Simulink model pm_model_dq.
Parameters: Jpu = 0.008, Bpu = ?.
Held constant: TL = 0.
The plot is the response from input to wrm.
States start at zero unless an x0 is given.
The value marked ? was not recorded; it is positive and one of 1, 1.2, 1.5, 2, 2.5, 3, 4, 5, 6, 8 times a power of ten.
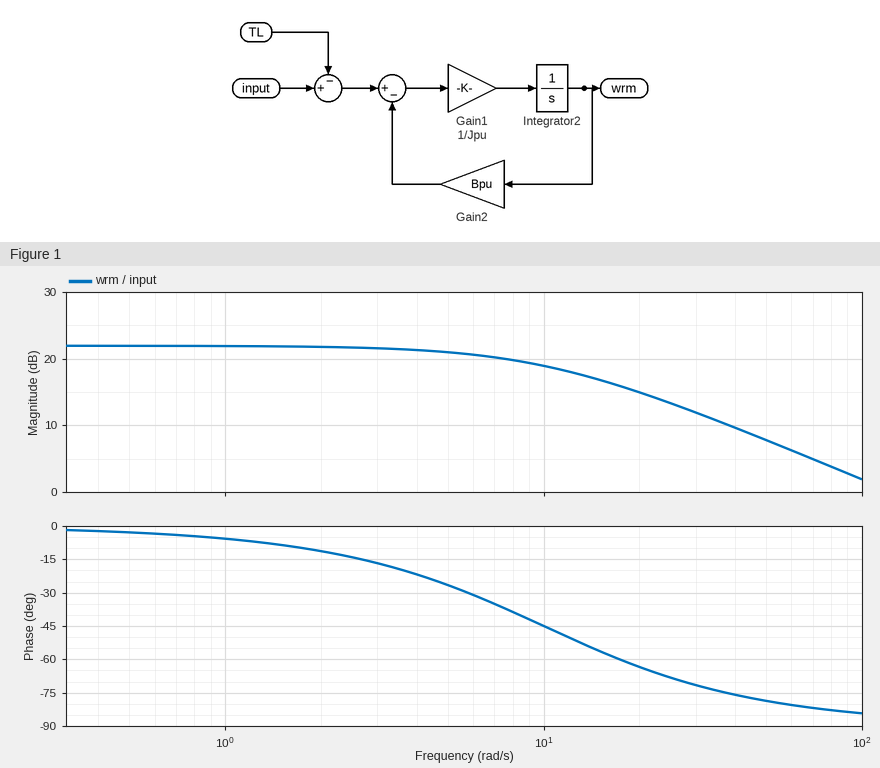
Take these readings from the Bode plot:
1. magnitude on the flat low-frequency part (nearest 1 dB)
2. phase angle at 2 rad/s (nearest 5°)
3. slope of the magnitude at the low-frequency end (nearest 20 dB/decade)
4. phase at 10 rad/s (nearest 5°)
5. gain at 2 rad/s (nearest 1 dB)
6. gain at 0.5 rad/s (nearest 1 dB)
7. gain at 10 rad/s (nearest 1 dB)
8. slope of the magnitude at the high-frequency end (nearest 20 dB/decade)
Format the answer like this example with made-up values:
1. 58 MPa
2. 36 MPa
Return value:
1. 22 dB
2. -10°
3. 0 dB/decade
4. -45°
5. 22 dB
6. 22 dB
7. 19 dB
8. -20 dB/decade
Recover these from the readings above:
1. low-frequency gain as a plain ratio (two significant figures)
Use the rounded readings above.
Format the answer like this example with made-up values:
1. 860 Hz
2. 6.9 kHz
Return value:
1. 13
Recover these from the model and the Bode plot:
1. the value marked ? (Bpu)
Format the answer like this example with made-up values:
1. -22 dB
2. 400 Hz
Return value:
1. 0.08
